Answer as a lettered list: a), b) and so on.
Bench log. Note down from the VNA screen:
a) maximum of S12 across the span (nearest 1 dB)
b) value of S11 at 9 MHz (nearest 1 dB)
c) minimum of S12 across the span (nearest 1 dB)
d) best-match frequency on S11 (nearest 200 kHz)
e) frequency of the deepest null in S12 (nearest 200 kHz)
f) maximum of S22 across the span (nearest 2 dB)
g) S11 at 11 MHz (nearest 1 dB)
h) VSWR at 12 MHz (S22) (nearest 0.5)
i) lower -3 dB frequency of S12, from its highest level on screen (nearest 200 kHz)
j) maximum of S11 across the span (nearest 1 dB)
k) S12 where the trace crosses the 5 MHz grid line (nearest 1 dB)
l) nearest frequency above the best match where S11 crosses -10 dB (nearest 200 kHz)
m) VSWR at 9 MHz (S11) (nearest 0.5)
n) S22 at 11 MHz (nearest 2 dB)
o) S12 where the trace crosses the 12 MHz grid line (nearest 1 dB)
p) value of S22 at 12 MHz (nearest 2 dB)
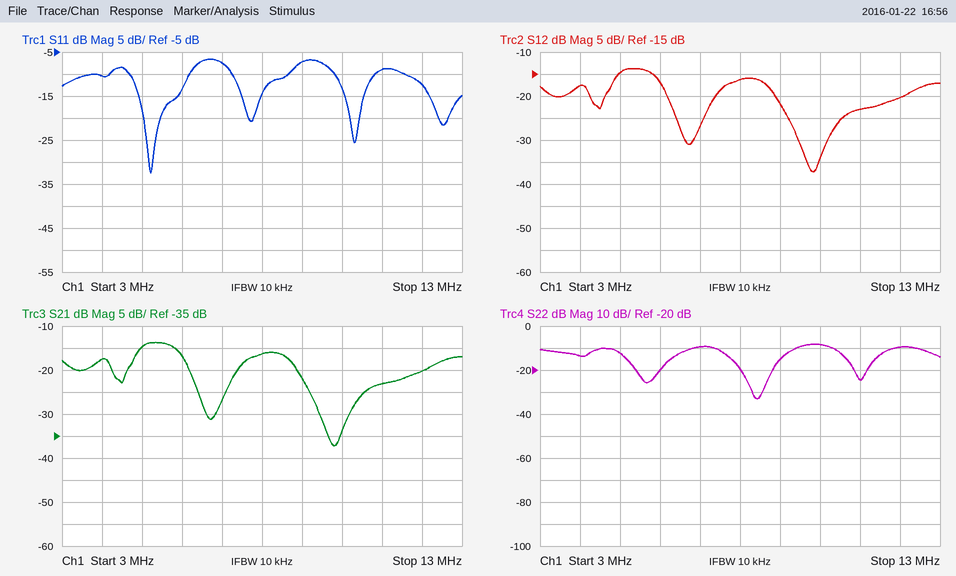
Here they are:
a) -14 dB
b) -7 dB
c) -37 dB
d) 5.2 MHz
e) 9.8 MHz
f) -8 dB
g) -9 dB
h) 2.0
i) 4.8 MHz
j) -7 dB
k) -15 dB
l) 6.2 MHz
m) 2.5
n) -24 dB
o) -20 dB
p) -10 dB
